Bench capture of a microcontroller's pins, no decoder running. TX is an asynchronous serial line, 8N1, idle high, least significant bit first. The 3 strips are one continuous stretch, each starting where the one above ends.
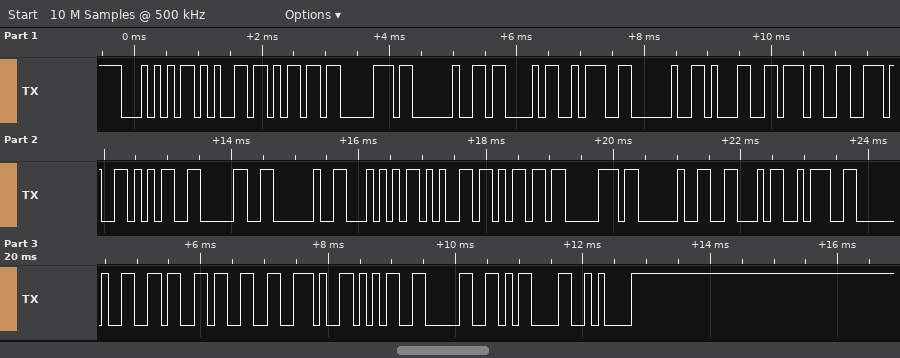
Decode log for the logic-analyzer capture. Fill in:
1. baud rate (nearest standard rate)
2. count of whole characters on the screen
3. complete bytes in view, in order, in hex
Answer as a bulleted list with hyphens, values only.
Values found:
- 9600 baud
- 29
- 54 65 6D 70 20 43 3A 20 31 37 2E 35 30 20 54 65 6D 70 20 46 3A 20 36 33 2E 35 30 0D 0A
